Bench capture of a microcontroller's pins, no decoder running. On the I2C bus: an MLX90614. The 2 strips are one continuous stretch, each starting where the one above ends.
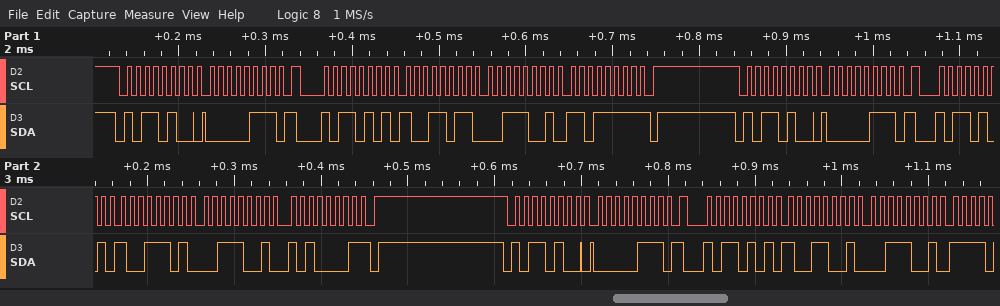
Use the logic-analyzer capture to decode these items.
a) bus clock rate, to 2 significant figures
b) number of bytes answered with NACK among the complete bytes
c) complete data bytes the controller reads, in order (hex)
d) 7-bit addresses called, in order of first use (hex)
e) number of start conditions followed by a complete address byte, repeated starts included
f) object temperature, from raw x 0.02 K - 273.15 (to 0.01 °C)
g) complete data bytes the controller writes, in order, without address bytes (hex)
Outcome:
100 kHz
2
9B 39 DF 9D 39 A1 99 39
0x5A
6
21.79 °C
07 07 07
